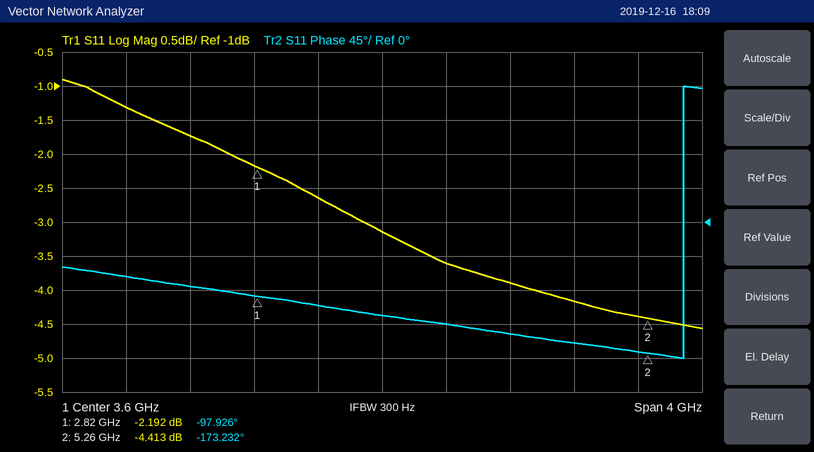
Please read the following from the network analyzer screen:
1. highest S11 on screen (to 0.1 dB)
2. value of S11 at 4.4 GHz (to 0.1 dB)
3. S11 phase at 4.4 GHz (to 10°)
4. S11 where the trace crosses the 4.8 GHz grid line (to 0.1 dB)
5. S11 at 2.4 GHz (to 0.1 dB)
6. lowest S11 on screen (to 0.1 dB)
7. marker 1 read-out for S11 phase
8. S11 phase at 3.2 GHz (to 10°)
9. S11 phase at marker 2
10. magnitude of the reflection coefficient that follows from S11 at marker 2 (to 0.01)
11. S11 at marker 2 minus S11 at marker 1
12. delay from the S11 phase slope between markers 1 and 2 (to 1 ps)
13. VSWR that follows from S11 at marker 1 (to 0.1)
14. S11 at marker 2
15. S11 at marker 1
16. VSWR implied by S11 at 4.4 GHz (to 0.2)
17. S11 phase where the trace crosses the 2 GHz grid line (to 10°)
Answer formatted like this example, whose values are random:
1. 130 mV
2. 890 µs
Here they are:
1. -0.9 dB
2. -3.9 dB
3. -150°
4. -4.2 dB
5. -1.7 dB
6. -4.6 dB
7. -97.926°
8. -110°
9. -173.232°
10. 0.60
11. -2.221 dB
12. 86 ps
13. 8.0
14. -4.413 dB
15. -2.192 dB
16. 4.6
17. -70°
